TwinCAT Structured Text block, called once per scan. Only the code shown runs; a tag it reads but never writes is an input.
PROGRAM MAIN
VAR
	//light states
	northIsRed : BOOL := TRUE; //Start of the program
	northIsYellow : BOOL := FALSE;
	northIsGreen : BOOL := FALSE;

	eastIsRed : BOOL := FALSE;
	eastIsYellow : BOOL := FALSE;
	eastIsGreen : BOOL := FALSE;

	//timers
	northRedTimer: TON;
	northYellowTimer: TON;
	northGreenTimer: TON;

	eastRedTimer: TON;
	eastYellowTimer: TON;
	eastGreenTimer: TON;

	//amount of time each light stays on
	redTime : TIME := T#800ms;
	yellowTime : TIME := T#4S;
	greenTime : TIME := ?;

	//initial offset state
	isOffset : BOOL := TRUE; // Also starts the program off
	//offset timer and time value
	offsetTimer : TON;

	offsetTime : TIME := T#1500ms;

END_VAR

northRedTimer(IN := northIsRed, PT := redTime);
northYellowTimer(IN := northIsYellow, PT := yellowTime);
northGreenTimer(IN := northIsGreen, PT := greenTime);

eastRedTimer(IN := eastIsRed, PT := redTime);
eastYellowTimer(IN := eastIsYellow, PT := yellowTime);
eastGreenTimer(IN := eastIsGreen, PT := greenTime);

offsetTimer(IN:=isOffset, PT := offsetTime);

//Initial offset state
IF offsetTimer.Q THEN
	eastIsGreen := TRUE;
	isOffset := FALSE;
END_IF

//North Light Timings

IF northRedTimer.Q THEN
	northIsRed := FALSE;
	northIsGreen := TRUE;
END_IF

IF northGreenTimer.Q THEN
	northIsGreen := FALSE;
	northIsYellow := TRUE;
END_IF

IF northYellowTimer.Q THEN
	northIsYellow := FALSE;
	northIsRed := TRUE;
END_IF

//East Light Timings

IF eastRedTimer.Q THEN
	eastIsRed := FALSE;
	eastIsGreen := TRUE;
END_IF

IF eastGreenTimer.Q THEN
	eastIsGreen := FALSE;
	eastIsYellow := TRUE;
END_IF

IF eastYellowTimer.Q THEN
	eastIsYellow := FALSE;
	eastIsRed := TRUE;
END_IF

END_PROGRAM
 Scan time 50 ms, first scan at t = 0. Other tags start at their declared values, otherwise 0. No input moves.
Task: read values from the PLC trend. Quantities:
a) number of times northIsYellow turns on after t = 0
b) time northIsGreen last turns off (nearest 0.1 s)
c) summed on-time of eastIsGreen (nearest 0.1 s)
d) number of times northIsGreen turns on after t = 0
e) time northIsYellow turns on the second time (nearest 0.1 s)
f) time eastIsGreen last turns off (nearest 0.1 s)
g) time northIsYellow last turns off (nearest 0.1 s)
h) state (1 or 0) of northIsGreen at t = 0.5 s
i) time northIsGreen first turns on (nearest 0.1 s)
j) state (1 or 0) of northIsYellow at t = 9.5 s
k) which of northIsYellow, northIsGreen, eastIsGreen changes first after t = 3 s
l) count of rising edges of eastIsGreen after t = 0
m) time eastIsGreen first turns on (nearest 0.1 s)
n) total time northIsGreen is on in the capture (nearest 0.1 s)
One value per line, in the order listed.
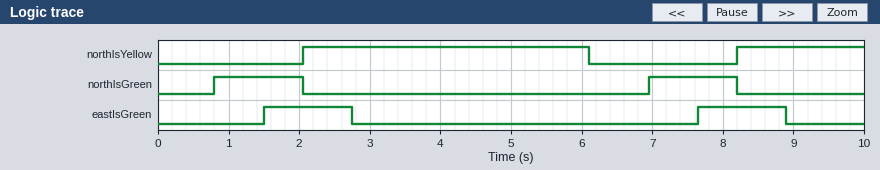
2
8.2 s
2.5 s
2
8.2 s
8.9 s
6.1 s
0
0.8 s
1
northIsYellow
2
1.5 s
2.5 s
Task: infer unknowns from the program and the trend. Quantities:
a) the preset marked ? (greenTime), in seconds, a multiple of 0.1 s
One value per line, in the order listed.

1.2 s
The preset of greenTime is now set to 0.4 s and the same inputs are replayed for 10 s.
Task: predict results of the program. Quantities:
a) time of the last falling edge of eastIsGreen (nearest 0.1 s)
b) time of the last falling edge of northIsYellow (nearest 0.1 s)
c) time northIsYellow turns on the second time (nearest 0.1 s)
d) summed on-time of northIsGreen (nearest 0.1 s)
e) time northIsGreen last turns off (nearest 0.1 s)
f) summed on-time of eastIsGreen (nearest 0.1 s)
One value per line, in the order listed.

7.3 s
5.3 s
6.6 s
0.9 s
6.6 s
0.9 s
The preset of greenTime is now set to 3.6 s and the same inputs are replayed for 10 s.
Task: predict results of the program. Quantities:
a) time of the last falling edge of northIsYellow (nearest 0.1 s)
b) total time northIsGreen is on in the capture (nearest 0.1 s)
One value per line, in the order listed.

8.5 s
4.3 s
